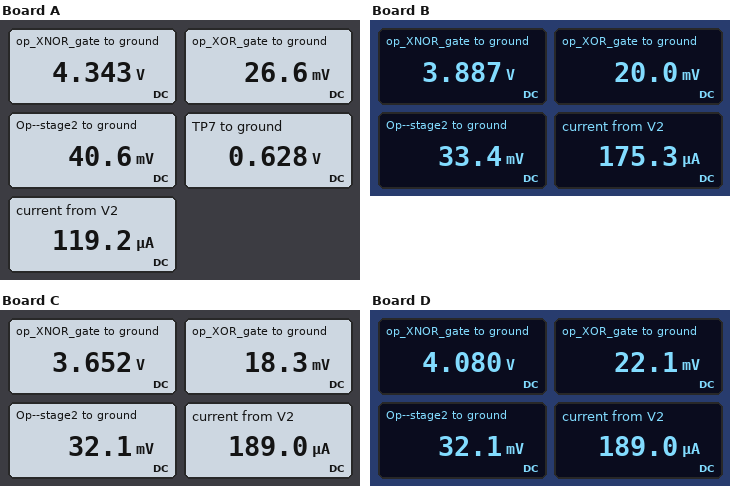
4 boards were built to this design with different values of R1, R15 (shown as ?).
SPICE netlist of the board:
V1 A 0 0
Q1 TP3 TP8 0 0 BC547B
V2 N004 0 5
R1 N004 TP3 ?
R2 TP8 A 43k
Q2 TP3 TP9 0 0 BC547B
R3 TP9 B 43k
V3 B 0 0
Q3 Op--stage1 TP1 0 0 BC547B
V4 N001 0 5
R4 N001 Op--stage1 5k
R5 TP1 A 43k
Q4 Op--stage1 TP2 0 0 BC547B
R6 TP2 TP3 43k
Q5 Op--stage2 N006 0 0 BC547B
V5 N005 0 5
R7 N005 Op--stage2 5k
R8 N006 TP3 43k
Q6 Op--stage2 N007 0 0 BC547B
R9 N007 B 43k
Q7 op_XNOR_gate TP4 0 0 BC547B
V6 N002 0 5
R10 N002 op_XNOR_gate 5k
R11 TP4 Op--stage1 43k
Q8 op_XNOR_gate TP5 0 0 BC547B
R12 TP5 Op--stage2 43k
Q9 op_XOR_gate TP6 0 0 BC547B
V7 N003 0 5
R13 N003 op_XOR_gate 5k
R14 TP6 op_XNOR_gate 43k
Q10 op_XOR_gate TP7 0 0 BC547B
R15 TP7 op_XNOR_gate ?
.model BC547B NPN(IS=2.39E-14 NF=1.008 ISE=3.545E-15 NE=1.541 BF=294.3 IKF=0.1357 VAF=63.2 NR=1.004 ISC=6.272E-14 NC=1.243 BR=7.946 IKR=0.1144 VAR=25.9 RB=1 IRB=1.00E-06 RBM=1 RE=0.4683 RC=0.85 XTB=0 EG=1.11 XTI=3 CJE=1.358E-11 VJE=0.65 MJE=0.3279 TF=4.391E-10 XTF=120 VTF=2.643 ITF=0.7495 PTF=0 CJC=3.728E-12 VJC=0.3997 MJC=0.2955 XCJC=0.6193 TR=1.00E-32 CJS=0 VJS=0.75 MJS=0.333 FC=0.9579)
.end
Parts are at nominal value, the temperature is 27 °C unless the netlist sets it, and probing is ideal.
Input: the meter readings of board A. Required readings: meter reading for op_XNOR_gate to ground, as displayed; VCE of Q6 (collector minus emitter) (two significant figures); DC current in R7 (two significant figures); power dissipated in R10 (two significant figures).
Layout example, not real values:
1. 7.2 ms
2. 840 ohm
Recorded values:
1. 4.343 V
2. 41 mV
3. 990 µA
4. 86 µW
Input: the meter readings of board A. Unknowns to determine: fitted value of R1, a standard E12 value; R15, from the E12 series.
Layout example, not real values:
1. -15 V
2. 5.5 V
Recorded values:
1. 15 kΩ
2. 82 kΩ
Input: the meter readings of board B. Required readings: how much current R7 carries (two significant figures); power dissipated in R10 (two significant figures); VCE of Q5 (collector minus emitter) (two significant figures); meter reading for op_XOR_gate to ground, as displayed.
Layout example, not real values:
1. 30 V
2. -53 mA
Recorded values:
1. 990 µA
2. 250 µW
3. 33 mV
4. 20.0 mV
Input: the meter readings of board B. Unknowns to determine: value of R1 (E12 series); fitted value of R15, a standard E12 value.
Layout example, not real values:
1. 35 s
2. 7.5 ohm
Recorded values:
1. 3.3 kΩ
2. 22 kΩ
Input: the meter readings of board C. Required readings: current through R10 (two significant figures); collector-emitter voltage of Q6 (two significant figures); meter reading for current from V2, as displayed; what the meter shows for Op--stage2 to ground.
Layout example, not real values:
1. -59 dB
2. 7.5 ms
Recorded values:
1. 270 µA
2. 32 mV
3. 189.0 µA
4. 32.1 mV
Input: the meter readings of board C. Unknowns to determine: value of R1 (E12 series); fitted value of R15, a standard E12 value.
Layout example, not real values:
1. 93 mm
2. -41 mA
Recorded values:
1. 1.5 kΩ
2. 15 kΩ
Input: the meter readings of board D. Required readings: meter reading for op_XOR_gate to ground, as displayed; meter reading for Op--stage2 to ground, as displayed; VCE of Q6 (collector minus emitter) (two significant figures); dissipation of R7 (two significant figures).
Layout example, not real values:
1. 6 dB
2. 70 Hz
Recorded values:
1. 22.1 mV
2. 32.1 mV
3. 32 mV
4. 4.9 mW
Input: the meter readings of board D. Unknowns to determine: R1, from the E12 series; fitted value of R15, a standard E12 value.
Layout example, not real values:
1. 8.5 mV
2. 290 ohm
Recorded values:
1. 1.5 kΩ
2. 33 kΩ
